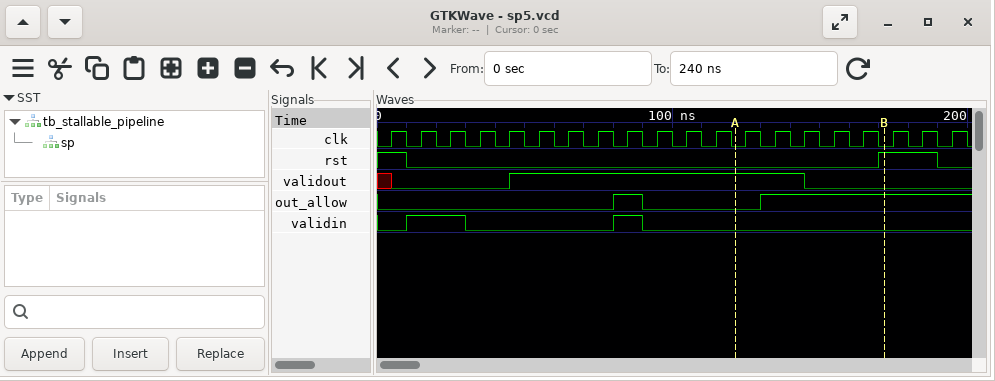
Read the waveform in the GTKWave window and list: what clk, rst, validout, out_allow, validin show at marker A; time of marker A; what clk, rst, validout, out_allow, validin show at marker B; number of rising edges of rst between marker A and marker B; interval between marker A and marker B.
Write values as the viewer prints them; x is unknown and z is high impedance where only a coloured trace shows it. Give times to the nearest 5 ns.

clk=0, rst=0, validout=1, out_allow=0, validin=0
120 ns
clk=0, rst=1, validout=0, out_allow=1, validin=0
1
50 ns
